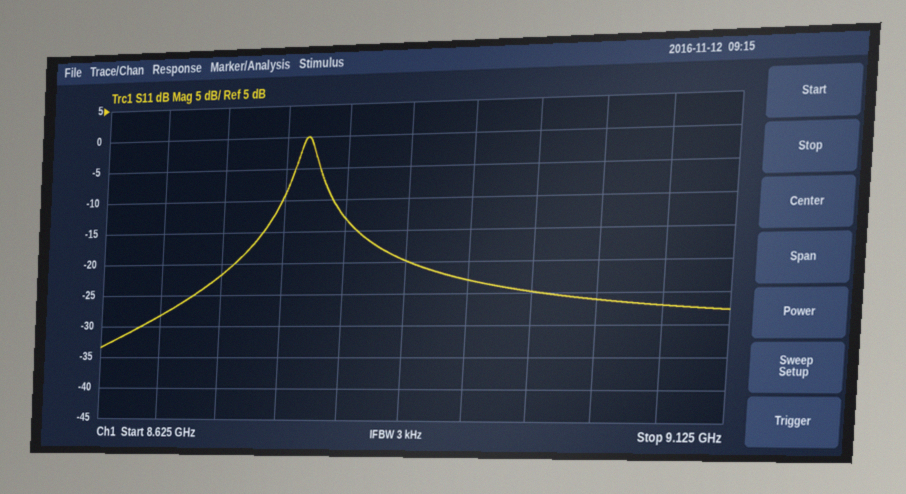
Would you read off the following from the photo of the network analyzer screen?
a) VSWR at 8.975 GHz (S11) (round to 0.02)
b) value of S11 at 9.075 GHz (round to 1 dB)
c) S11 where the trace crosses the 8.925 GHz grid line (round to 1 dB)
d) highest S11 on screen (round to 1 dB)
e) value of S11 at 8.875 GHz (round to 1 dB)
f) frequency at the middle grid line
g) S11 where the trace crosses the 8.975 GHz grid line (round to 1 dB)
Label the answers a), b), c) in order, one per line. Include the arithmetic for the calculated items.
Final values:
a) |Γ| = 10^(-25/20) = 0.0562; VSWR = (1 + 0.0562)/(1 − 0.0562) ≈ 1.12
b) -27 dB
c) -23 dB
d) 0 dB
e) -20 dB
f) 8.875 GHz
g) -25 dB
